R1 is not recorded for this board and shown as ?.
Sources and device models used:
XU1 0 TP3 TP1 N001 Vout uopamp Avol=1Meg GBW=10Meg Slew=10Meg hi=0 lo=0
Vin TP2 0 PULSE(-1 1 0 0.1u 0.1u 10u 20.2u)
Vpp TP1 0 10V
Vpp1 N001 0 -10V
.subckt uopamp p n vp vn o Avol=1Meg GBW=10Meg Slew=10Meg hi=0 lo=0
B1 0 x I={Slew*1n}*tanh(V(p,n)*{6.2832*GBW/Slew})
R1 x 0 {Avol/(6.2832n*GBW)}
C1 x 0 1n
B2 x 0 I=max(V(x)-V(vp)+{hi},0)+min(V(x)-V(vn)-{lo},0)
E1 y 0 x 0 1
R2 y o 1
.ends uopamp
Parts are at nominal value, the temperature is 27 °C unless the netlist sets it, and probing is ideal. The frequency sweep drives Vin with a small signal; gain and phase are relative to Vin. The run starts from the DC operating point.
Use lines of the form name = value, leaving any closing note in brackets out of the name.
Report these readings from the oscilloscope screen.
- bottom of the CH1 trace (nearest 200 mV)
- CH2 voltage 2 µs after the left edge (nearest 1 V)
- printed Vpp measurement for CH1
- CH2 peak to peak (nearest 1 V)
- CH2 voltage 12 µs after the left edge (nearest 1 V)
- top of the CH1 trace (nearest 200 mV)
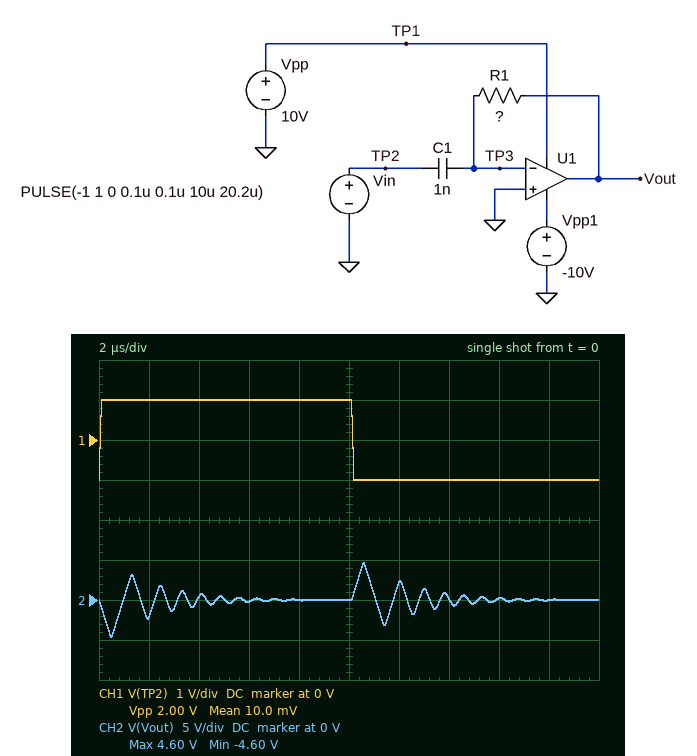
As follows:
bottom of the CH1 trace = -1.0 V
CH2 voltage 2 µs after the left edge = -2 V
printed Vpp measurement for CH1 = 2.00 V
CH2 peak to peak = 9 V
CH2 voltage 12 µs after the left edge = 2 V
top of the CH1 trace = 1.0 V
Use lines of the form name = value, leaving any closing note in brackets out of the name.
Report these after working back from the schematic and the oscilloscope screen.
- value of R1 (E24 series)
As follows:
value of R1 = 820 Ω
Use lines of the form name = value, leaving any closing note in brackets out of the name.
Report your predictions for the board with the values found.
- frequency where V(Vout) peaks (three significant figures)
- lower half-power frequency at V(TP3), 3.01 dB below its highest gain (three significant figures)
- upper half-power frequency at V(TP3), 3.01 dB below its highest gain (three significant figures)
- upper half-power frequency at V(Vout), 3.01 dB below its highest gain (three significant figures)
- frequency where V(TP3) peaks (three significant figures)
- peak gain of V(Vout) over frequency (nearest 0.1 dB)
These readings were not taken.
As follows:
frequency where V(Vout) peaks = 1.39 MHz
lower half-power frequency at V(TP3), 3.01 dB below its highest gain = 1.31 MHz
upper half-power frequency at V(TP3), 3.01 dB below its highest gain = 1.51 MHz
upper half-power frequency at V(Vout), 3.01 dB below its highest gain = 1.49 MHz
frequency where V(TP3) peaks = 1.40 MHz
peak gain of V(Vout) over frequency = 34.2 dB
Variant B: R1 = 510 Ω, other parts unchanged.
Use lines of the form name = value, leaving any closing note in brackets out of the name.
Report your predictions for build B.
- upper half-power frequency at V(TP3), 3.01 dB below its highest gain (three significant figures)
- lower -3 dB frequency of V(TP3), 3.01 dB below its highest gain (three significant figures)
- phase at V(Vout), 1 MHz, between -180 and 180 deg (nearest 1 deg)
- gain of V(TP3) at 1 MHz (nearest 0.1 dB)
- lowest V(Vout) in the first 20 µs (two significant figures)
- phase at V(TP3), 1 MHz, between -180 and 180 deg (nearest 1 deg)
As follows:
upper half-power frequency at V(TP3), 3.01 dB below its highest gain = 1.96 MHz
lower -3 dB frequency of V(TP3), 3.01 dB below its highest gain = 1.64 MHz
phase at V(Vout), 1 MHz, between -180 and 180 deg = -98 deg
gain of V(TP3) at 1 MHz = -6.6 dB
lowest V(Vout) in the first 20 µs = -3.5 V
phase at V(TP3), 1 MHz, between -180 and 180 deg = 172 deg
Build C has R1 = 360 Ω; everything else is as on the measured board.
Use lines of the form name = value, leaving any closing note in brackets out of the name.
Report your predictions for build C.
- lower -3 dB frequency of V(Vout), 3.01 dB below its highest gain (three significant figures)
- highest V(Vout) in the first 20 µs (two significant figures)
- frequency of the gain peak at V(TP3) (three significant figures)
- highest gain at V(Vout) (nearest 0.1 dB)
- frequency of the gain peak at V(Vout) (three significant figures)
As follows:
lower -3 dB frequency of V(Vout), 3.01 dB below its highest gain = 1.89 MHz
highest V(Vout) in the first 20 µs = 2.9 V
frequency of the gain peak at V(TP3) = 2.12 MHz
highest gain at V(Vout) = 27.1 dB
frequency of the gain peak at V(Vout) = 2.10 MHz
